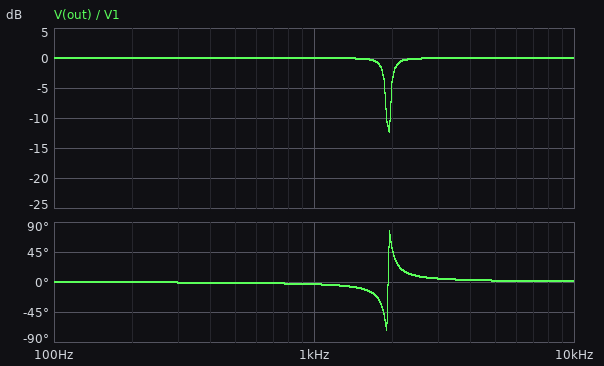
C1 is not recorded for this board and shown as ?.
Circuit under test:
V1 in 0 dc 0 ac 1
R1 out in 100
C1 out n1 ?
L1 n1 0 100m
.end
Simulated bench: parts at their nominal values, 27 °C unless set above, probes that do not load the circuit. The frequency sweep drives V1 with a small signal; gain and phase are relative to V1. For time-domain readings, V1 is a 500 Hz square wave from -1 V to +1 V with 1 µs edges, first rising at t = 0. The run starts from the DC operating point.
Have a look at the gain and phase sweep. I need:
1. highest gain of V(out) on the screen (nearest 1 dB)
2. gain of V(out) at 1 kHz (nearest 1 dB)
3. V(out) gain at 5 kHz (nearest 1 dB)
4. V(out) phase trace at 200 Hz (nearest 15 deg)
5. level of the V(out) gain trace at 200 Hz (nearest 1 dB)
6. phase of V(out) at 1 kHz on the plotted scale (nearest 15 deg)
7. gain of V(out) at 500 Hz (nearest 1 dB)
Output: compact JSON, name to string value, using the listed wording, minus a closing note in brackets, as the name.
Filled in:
{"highest gain of V(out) on the screen": "0 dB", "gain of V(out) at 1 kHz": "0 dB", "V(out) gain at 5 kHz": "0 dB", "V(out) phase trace at 200 Hz": "0 deg", "level of the V(out) gain trace at 200 Hz": "0 dB", "phase of V(out) at 1 kHz on the plotted scale": "0 deg", "gain of V(out) at 500 Hz": "0 dB"}
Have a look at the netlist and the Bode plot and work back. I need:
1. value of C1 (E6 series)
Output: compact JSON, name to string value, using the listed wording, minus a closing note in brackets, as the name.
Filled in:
{"value of C1": "68 nF"}
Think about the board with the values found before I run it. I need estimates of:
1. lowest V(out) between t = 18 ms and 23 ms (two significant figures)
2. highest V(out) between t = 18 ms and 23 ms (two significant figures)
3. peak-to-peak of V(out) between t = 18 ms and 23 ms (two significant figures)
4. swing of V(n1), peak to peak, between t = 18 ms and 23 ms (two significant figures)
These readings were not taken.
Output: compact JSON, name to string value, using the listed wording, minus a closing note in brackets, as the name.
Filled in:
{"lowest V(out) between t = 18 ms and 23 ms": "-1.1 V", "highest V(out) between t = 18 ms and 23 ms": "1.1 V", "peak-to-peak of V(out) between t = 18 ms and 23 ms": "2.2 V", "swing of V(n1), peak to peak, between t = 18 ms and 23 ms": "2.5 V"}
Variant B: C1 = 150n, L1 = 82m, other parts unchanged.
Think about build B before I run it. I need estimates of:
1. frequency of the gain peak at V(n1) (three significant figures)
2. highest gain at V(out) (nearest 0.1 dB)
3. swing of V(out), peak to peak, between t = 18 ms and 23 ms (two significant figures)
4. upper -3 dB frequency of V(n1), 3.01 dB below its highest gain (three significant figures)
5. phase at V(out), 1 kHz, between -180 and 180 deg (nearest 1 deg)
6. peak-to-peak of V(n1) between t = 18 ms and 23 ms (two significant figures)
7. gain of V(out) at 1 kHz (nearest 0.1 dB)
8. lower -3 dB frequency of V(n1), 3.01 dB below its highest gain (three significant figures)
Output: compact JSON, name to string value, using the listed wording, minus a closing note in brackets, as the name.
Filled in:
{"frequency of the gain peak at V(n1)": "1.44 kHz", "highest gain at V(out)": "0 dB", "swing of V(out), peak to peak, between t = 18 ms and 23 ms": "2.7 V", "upper -3 dB frequency of V(n1), 3.01 dB below its highest gain": "1.55 kHz", "phase at V(out), 1 kHz, between -180 and 180 deg": "-10 deg", "peak-to-peak of V(n1) between t = 18 ms and 23 ms": "7.1 V", "gain of V(out) at 1 kHz": "-0.1 dB", "lower -3 dB frequency of V(n1), 3.01 dB below its highest gain": "1.35 kHz"}
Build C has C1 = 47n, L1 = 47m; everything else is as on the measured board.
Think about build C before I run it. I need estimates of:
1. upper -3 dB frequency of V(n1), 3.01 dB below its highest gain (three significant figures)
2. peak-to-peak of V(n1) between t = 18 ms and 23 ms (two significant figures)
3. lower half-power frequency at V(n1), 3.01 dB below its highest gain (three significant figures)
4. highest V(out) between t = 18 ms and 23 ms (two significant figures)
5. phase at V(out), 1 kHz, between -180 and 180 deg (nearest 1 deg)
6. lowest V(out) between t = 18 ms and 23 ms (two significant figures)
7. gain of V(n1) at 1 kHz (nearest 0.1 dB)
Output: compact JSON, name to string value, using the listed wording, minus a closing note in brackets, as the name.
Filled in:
{"upper -3 dB frequency of V(n1), 3.01 dB below its highest gain": "3.58 kHz", "peak-to-peak of V(n1) between t = 18 ms and 23 ms": "5.0 V", "lower half-power frequency at V(n1), 3.01 dB below its highest gain": "3.24 kHz", "highest V(out) between t = 18 ms and 23 ms": "1.2 V", "phase at V(out), 1 kHz, between -180 and 180 deg": "-2 deg", "lowest V(out) between t = 18 ms and 23 ms": "-1.2 V", "gain of V(n1) at 1 kHz": "-20.4 dB"}
